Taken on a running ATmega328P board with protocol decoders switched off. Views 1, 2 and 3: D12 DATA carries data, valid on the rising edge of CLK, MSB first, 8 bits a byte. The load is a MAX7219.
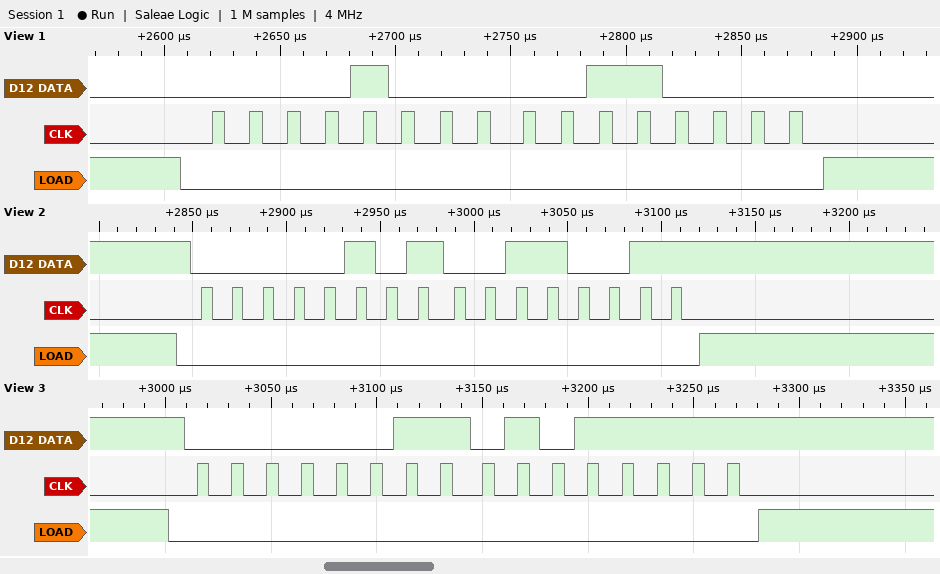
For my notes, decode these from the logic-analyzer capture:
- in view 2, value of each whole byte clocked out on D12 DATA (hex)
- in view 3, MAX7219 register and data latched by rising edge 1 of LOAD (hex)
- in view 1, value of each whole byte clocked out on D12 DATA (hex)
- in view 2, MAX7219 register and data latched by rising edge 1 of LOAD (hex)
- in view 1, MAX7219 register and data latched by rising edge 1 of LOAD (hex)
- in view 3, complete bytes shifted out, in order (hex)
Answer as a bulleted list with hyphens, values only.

- 0x05 0x33
- register 0x3, data 0x5F
- 0x08 0x30
- register 0x5, data 0x33
- register 0x8, data 0x30
- 03 5F
